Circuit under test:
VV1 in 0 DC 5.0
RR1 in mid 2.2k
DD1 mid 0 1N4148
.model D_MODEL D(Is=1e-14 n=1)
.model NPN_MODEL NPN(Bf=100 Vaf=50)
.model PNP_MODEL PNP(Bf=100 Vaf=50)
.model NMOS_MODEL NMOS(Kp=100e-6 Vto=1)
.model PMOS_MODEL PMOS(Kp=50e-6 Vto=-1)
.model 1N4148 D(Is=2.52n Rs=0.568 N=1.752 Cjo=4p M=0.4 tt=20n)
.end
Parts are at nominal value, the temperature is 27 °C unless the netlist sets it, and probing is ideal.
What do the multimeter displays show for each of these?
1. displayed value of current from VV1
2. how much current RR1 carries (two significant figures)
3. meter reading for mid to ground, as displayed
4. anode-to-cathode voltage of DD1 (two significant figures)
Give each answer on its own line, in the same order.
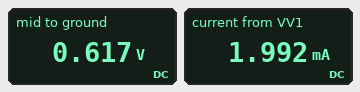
1.992 mA
2.0 mA
0.617 V
620 mV
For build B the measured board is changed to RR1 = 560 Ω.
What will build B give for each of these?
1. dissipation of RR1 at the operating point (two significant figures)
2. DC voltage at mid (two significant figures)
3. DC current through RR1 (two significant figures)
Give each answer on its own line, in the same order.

33 mW
680 mV
7.7 mA
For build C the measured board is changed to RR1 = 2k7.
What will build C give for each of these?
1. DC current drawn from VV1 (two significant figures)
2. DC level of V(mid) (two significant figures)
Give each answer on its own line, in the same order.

1.6 mA
610 mV
